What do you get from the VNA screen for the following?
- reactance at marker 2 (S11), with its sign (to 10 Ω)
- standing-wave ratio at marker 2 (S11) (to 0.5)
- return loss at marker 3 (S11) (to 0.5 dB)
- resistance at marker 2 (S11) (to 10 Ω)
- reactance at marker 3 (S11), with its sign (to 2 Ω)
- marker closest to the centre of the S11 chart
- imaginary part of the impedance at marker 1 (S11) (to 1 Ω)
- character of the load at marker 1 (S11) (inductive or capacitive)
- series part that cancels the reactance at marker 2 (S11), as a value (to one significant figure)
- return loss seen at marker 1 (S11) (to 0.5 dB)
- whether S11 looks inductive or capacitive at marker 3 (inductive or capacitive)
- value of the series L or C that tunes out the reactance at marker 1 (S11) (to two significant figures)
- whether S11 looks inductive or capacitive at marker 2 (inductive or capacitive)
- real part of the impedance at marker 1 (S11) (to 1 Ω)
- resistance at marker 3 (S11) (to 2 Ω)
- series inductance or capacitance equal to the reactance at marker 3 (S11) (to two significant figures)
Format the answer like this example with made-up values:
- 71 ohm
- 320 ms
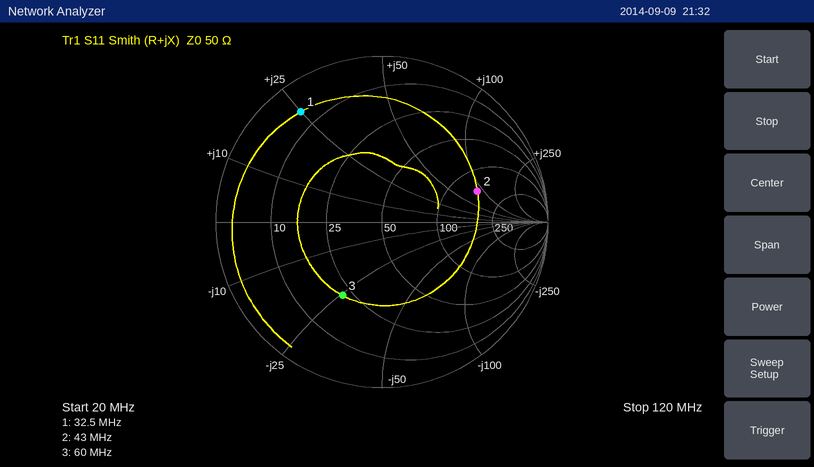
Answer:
- +90 Ω
- 4.0
- 6.0 dB
- 150 Ω
- -26 Ω
- marker 3
- +25 Ω
- inductive
- 40 pF
- 1.5 dB
- capacitive
- 200 pF
- inductive
- 6 Ω
- 22 Ω
- 100 pF
